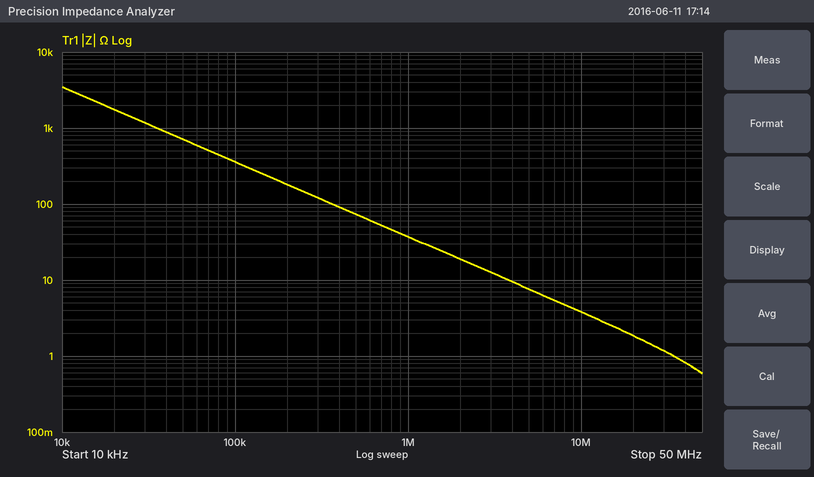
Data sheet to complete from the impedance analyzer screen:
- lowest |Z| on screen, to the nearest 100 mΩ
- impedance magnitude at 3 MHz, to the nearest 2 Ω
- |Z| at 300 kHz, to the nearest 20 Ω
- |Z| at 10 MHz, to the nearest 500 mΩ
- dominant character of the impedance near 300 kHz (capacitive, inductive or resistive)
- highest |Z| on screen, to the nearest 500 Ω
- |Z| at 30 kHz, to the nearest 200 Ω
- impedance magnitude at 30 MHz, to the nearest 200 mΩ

600 mΩ
12 Ω
120 Ω
4.0 Ω
capacitive
3.5 kΩ
1.2 kΩ
1.2 Ω
